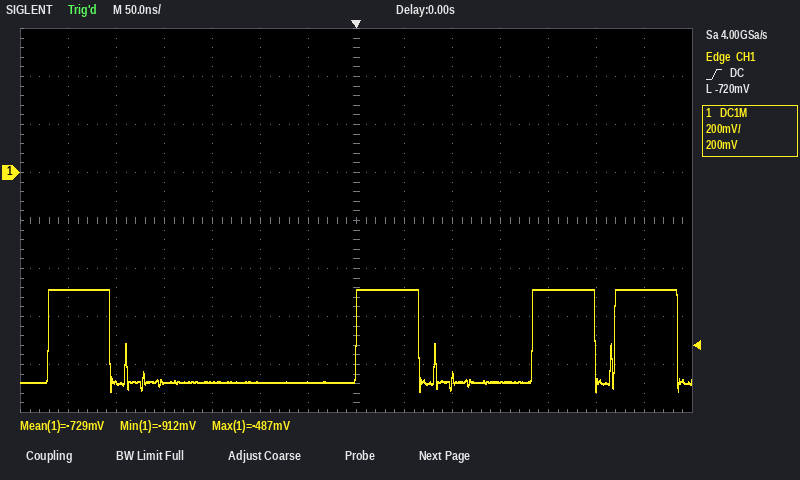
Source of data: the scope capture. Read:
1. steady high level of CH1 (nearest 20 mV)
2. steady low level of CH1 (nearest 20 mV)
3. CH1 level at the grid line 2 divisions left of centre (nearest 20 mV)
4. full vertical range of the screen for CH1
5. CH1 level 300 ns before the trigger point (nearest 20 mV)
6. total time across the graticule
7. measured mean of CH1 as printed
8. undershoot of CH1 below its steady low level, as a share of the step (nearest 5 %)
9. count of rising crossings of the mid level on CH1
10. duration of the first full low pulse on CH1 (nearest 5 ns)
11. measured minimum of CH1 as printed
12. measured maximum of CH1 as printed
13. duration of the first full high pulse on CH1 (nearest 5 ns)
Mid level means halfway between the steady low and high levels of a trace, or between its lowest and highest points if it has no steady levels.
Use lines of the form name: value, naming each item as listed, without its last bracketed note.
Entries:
steady high level of CH1: -480 mV
steady low level of CH1: -880 mV
CH1 level at the grid line 2 divisions left of centre: -880 mV
full vertical range of the screen for CH1: 1.6 V
CH1 level 300 ns before the trigger point: -480 mV
total time across the graticule: 700 ns
measured mean of CH1 as printed: -729 mV
undershoot of CH1 below its steady low level, as a share of the step: 10 %
count of rising crossings of the mid level on CH1: 4
duration of the first full low pulse on CH1: 255 ns
measured minimum of CH1 as printed: -912 mV
measured maximum of CH1 as printed: -487 mV
duration of the first full high pulse on CH1: 65 ns
